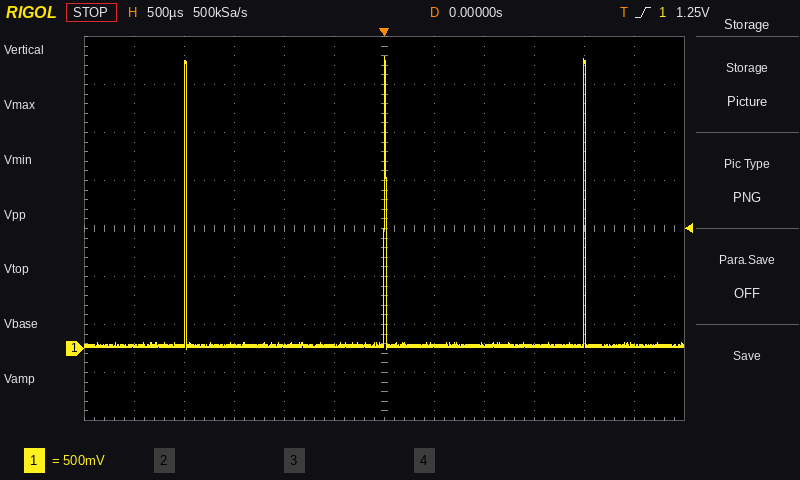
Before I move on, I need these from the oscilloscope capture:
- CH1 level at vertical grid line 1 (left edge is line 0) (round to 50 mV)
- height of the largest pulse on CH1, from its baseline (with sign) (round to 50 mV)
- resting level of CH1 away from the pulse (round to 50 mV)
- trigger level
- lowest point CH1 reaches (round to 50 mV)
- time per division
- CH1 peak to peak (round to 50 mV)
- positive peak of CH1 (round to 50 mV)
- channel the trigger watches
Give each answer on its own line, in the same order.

50 mV
+3.00 V
50 mV
1.25 V
0 mV
500 µs
3.05 V
3.05 V
CH1
